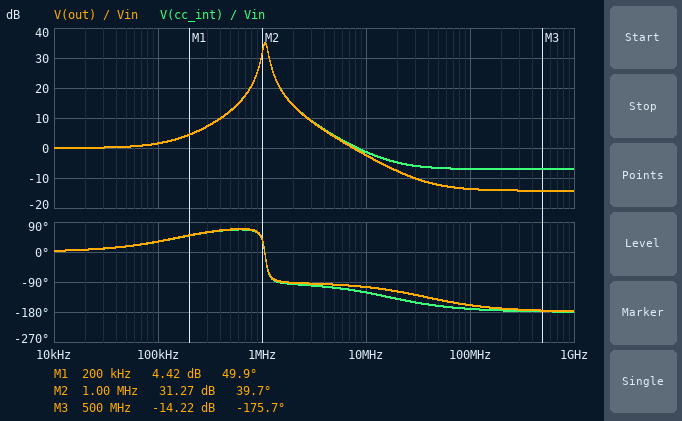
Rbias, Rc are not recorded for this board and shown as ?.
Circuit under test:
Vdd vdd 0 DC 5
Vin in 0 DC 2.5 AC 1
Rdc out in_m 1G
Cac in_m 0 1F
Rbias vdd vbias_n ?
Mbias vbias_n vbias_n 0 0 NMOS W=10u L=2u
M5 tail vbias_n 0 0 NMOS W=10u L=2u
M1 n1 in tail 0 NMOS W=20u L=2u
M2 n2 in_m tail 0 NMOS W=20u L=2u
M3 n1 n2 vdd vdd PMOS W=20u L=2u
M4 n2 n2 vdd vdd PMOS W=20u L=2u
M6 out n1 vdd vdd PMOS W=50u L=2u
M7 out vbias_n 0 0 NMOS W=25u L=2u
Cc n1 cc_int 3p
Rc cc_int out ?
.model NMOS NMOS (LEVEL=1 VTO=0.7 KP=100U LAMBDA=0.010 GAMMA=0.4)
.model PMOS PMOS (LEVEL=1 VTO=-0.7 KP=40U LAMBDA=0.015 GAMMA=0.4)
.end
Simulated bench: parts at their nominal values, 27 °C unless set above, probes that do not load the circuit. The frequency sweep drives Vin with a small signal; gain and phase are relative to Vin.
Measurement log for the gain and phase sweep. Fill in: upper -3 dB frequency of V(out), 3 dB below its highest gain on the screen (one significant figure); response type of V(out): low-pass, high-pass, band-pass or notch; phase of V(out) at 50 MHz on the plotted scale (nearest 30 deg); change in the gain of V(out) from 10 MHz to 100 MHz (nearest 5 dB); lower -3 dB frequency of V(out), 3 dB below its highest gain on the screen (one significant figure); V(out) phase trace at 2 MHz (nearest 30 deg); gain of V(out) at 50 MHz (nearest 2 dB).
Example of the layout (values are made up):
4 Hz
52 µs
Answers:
1 MHz
band-pass
-150 deg
-10 dB
1 MHz
-90 deg
-12 dB
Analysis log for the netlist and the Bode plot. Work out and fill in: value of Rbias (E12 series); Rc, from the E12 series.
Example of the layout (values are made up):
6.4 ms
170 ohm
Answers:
220 kΩ
1.8 kΩ
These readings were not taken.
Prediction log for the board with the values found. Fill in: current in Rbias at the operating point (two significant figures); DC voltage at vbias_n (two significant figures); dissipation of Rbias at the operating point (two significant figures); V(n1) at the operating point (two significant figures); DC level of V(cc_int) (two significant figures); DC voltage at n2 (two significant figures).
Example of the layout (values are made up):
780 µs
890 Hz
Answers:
18 µA
970 mV
74 µW
4.0 V
2.5 V
4.1 V
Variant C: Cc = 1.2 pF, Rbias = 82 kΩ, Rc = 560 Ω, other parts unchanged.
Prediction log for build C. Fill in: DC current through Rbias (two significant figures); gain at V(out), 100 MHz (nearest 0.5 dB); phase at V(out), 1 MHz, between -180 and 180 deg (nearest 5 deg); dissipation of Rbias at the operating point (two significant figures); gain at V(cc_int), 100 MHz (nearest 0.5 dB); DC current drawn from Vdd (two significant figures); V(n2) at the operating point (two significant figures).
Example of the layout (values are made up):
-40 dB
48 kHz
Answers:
47 µA
-7.5 dB
80 deg
180 µW
-5.5 dB
210 µA
4.0 V
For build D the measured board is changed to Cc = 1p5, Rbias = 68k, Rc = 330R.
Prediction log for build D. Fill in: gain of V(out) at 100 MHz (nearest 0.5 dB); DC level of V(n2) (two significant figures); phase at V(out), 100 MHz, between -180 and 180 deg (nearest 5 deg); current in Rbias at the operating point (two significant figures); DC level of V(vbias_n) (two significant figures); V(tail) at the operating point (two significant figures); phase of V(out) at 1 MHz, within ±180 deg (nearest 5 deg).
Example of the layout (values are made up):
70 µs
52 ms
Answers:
-7.0 dB
3.9 V
-145 deg
56 µA
1.2 V
1.3 V
80 deg
